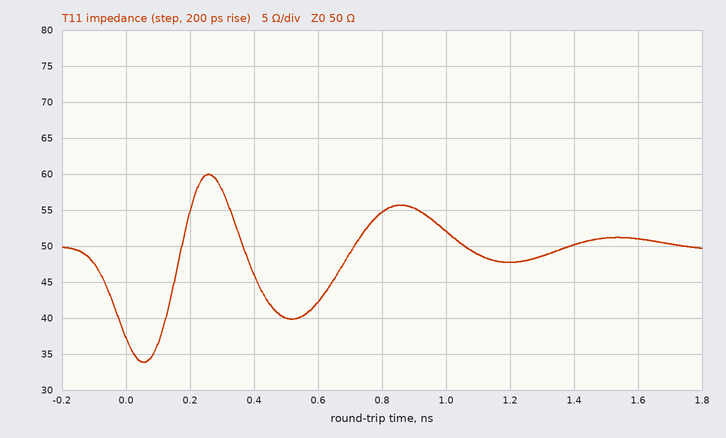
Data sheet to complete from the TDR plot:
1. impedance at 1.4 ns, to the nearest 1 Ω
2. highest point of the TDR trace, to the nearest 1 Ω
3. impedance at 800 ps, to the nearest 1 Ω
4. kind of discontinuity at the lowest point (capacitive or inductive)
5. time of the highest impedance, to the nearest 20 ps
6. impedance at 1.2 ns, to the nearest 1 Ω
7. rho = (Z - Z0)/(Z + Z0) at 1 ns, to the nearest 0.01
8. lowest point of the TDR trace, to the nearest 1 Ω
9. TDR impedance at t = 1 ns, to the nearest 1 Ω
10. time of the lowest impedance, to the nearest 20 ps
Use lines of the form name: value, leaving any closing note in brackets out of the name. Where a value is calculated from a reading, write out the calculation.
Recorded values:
impedance at 1.4 ns, to the nearest 1 Ω: 50 Ω
highest point of the TDR trace, to the nearest 1 Ω: 60 Ω
impedance at 800 ps, to the nearest 1 Ω: 55 Ω
kind of discontinuity at the lowest point: capacitive
time of the highest impedance, to the nearest 20 ps: 260 ps
impedance at 1.2 ns, to the nearest 1 Ω: 48 Ω
rho = (Z - Z0)/(Z + Z0) at 1 ns, to the nearest 0.01: (52 − 50)/(52 + 50) ≈ +0.02
lowest point of the TDR trace, to the nearest 1 Ω: 34 Ω
TDR impedance at t = 1 ns, to the nearest 1 Ω: 52 Ω
time of the lowest impedance, to the nearest 20 ps: 60 ps
